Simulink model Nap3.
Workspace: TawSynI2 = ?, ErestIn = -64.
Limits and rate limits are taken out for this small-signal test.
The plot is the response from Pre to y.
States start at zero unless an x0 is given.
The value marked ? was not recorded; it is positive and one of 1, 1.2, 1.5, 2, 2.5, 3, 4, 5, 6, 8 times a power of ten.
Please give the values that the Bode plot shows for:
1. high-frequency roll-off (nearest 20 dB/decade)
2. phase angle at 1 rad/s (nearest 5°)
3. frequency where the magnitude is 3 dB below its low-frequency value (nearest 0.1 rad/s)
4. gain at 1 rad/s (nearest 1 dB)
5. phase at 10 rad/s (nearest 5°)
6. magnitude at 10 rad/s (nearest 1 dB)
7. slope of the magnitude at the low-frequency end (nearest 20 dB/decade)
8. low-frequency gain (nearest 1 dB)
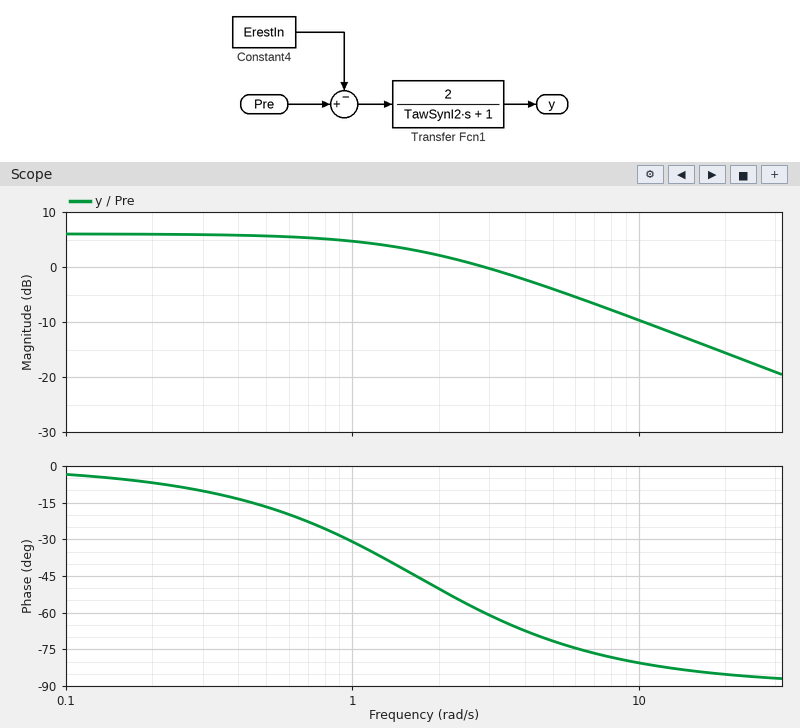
-20 dB/decade
-30°
1.7 rad/s
5 dB
-80°
-10 dB
0 dB/decade
6 dB
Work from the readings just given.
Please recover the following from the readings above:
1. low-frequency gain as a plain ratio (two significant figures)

2.0
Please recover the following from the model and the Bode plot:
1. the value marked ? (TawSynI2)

0.6
